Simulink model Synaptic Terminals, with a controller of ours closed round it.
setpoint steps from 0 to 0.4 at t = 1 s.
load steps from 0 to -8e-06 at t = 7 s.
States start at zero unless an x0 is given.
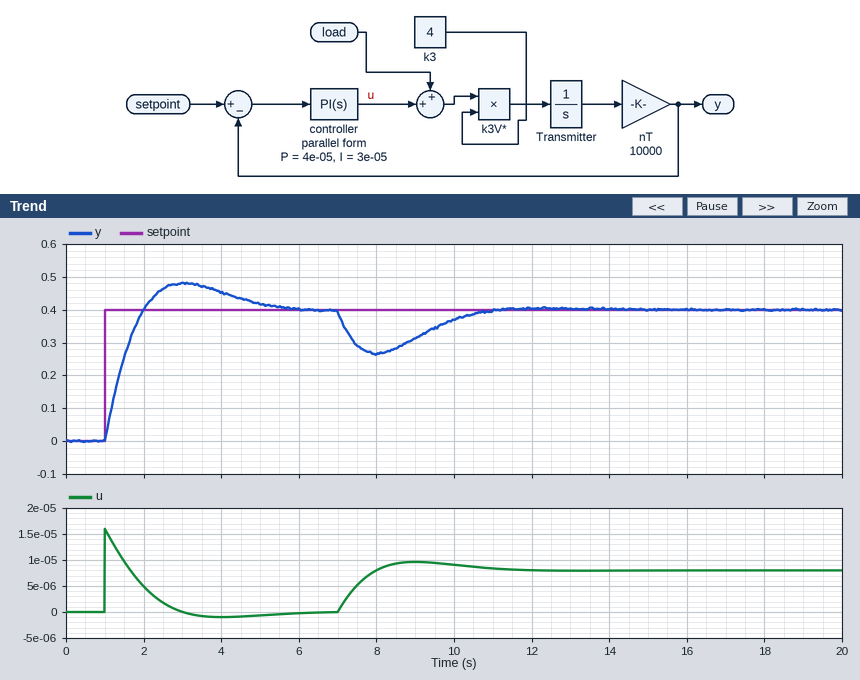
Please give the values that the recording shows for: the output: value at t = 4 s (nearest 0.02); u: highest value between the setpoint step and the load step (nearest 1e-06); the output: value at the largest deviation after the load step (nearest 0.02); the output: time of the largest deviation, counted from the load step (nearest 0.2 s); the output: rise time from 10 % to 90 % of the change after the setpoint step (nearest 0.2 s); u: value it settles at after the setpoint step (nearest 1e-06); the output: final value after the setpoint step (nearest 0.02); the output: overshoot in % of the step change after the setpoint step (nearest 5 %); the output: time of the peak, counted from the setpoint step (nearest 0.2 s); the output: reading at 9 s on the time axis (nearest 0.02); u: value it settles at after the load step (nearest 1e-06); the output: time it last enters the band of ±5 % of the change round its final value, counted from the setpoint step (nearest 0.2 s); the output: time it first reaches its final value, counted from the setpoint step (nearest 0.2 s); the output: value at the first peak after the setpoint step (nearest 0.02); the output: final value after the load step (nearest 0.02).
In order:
0.46
0.000016
0.26
1.0 s
0.8 s
0.000000
0.40
20 %
2.0 s
0.32
0.000008
4.0 s
1.0 s
0.48
0.40
